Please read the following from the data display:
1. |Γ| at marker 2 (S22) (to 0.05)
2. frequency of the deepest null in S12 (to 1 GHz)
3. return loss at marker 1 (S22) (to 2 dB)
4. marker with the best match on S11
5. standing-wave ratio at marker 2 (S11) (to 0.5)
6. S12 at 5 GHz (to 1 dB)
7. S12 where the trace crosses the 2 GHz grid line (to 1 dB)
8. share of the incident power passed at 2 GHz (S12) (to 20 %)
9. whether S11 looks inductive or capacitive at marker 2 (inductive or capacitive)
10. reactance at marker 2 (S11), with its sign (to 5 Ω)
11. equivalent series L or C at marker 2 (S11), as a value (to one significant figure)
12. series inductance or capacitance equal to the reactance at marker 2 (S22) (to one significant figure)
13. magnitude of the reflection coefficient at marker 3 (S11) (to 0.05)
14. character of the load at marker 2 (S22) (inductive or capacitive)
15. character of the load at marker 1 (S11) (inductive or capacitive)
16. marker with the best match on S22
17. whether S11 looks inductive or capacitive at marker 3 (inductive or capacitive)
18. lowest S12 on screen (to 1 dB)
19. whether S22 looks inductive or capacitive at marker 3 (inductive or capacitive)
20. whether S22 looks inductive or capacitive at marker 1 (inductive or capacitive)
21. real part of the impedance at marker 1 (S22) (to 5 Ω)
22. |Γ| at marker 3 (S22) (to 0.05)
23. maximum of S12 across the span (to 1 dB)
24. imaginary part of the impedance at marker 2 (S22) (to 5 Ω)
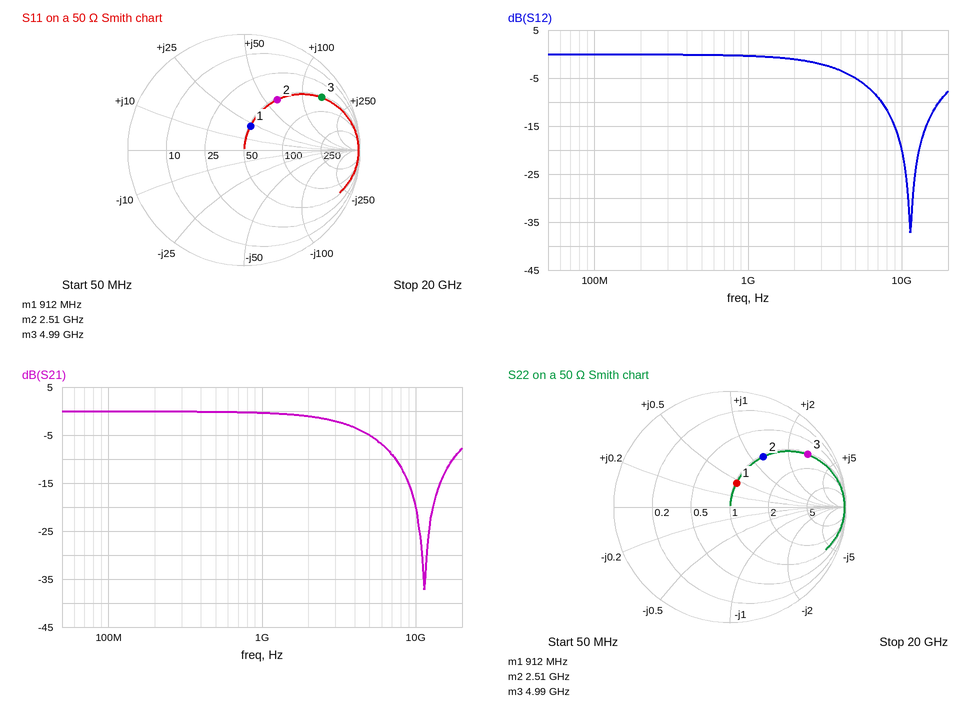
0.50
11 GHz
14 dB
marker 1
3.0
-5 dB
-1 dB
80 %
inductive
+60 Ω
4 nH
4 nH
0.80
inductive
inductive
marker 1
inductive
-37 dB
inductive
inductive
50 Ω
0.80
0 dB
+60 Ω
